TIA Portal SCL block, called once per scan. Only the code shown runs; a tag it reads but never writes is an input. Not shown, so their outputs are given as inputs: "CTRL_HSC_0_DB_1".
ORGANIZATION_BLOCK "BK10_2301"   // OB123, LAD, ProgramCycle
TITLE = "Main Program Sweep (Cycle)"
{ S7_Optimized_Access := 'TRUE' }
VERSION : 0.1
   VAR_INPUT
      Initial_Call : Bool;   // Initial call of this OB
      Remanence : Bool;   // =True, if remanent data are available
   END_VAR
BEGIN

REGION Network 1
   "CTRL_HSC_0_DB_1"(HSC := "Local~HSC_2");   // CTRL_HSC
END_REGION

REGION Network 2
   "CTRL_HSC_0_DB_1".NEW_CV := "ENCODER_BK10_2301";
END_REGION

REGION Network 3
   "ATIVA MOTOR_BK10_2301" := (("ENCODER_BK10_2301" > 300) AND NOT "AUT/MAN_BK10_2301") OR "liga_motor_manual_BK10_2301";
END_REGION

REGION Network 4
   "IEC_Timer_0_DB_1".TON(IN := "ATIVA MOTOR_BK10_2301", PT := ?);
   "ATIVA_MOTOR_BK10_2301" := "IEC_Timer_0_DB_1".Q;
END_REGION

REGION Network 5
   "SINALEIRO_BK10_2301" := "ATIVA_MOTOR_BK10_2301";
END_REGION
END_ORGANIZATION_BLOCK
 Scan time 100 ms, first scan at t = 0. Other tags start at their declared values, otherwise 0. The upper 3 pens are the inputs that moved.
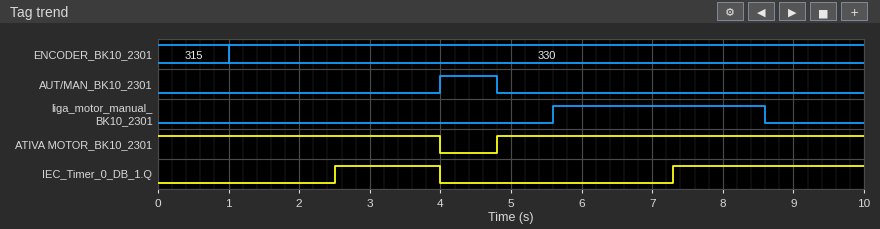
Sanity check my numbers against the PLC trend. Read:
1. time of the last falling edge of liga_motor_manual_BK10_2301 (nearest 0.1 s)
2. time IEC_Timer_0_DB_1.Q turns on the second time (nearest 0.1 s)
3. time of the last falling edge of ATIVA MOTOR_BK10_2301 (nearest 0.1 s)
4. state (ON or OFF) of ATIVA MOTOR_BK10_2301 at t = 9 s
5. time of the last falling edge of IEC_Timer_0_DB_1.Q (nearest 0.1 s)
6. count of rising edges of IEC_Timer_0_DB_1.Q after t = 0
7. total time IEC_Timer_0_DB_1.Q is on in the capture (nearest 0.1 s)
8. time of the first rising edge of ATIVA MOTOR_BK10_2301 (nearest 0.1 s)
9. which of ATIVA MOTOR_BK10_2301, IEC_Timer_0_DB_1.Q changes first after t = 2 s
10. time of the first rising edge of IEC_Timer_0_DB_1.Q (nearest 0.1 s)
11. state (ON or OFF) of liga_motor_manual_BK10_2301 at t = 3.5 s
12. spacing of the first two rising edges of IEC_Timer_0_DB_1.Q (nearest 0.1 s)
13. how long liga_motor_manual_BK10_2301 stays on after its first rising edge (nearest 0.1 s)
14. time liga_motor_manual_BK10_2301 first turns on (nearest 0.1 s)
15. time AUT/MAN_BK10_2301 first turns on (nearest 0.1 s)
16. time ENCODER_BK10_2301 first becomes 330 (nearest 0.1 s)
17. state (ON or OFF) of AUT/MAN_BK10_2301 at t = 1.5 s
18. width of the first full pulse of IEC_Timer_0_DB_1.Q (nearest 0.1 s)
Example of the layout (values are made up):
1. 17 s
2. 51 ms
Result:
1. 8.6 s
2. 7.3 s
3. 4.0 s
4. ON
5. 4.0 s
6. 2
7. 4.2 s
8. 4.8 s
9. IEC_Timer_0_DB_1.Q
10. 2.5 s
11. OFF
12. 4.8 s
13. 3.0 s
14. 5.6 s
15. 4.0 s
16. 1.0 s
17. OFF
18. 1.5 s
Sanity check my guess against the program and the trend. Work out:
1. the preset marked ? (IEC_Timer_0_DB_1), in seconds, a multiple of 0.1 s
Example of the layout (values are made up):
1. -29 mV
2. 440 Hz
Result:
1. 2.5 s
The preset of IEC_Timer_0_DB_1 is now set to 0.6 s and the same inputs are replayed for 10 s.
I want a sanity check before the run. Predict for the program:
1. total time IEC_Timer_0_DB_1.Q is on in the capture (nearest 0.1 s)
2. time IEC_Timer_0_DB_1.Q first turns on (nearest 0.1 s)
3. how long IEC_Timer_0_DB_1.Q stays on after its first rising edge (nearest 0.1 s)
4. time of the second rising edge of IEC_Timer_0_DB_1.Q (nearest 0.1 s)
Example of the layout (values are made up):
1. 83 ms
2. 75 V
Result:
1. 8.0 s
2. 0.6 s
3. 3.4 s
4. 5.4 s
